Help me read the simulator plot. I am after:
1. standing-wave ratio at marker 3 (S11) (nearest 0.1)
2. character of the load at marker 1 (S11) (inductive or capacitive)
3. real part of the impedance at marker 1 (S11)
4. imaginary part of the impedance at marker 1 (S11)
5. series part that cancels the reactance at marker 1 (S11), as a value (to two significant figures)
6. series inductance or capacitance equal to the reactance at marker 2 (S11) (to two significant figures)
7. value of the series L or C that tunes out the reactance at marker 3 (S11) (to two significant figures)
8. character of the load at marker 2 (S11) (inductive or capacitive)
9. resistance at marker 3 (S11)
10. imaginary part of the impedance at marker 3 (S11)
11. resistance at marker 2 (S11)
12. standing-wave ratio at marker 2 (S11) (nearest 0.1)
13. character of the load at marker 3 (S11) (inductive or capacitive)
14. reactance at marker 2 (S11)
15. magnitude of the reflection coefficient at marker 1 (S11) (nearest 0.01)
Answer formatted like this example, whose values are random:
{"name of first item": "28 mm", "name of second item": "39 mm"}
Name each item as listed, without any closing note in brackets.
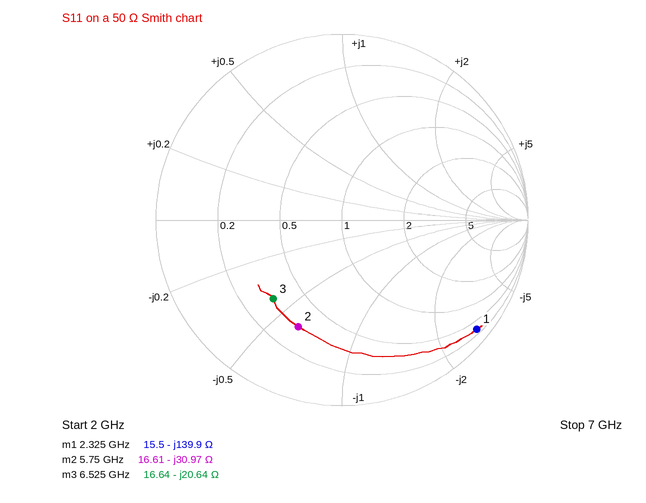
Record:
{"standing-wave ratio at marker 3 (S11)": "3.6", "character of the load at marker 1 (S11)": "capacitive", "real part of the impedance at marker 1": "15.5 Ω", "imaginary part of the impedance at marker 1": "-139.9 Ω", "series part that cancels the reactance at marker 1 (S11), as a value": "9.6 nH", "series inductance or capacitance equal to the reactance at marker 2 (S11)": "890 fF", "value of the series L or C that tunes out the reactance at marker 3 (S11)": "500 pH", "character of the load at marker 2 (S11)": "capacitive", "resistance at marker 3": "16.64 Ω", "imaginary part of the impedance at marker 3": "-20.64 Ω", "resistance at marker 2": "16.61 Ω", "standing-wave ratio at marker 2 (S11)": "4.3", "character of the load at marker 3 (S11)": "capacitive", "reactance at marker 2": "-30.97 Ω", "magnitude of the reflection coefficient at marker 1 (S11)": "0.93"}
